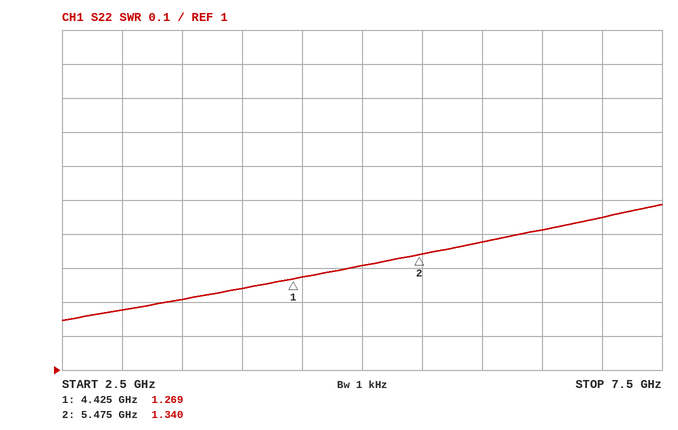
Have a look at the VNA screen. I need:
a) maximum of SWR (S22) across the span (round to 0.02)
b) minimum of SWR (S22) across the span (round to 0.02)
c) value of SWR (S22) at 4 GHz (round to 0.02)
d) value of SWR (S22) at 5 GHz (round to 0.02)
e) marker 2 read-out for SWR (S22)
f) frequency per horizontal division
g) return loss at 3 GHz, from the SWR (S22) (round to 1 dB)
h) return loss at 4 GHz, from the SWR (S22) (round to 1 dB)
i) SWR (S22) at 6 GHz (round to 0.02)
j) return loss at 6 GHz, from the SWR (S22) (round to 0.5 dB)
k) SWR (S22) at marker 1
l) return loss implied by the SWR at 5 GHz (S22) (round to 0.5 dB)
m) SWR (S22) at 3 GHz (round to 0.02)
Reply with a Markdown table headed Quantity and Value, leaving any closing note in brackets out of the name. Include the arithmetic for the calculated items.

| Quantity | Value |
|---|---|
| maximum of SWR (S22) across the span | 1.48 |
| minimum of SWR (S22) across the span | 1.14 |
| value of SWR (S22) at 4 GHz | 1.24 |
| value of SWR (S22) at 5 GHz | 1.30 |
| marker 2 read-out for SWR | 1.340 |
| frequency per horizontal division | 500 MHz |
| return loss at 3 GHz, from the SWR (S22) | −20 log10((1.18 − 1)/(1.18 + 1)) ≈ 22 dB |
| return loss at 4 GHz, from the SWR (S22) | −20 log10((1.24 − 1)/(1.24 + 1)) ≈ 19 dB |
| SWR (S22) at 6 GHz | 1.38 |
| return loss at 6 GHz, from the SWR (S22) | −20 log10((1.38 − 1)/(1.38 + 1)) ≈ 15.9 dB, so 16.0 dB to the nearest 0.5 dB |
| SWR (S22) at marker 1 | 1.269 |
| return loss implied by the SWR at 5 GHz (S22) | −20 log10((1.3 − 1)/(1.3 + 1)) ≈ 17.7 dB, so 17.5 dB to the nearest 0.5 dB |
| SWR (S22) at 3 GHz | 1.18 |
